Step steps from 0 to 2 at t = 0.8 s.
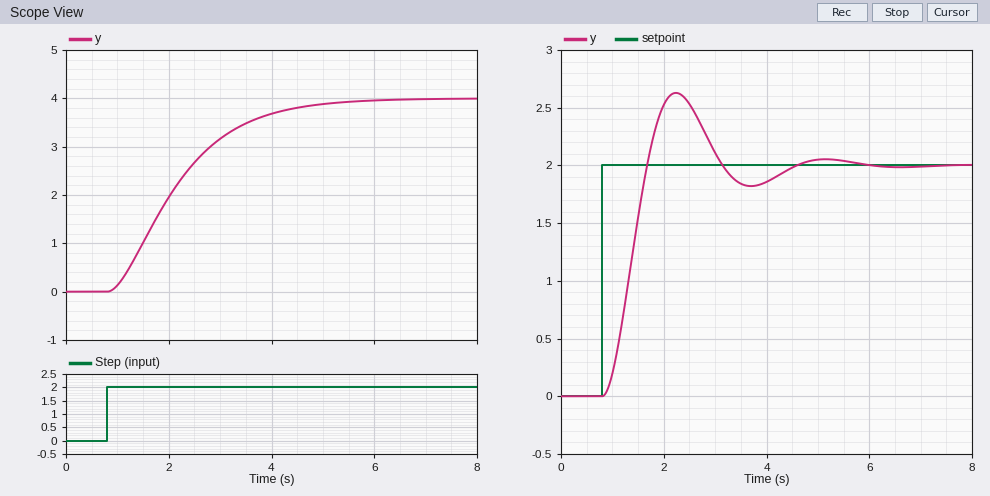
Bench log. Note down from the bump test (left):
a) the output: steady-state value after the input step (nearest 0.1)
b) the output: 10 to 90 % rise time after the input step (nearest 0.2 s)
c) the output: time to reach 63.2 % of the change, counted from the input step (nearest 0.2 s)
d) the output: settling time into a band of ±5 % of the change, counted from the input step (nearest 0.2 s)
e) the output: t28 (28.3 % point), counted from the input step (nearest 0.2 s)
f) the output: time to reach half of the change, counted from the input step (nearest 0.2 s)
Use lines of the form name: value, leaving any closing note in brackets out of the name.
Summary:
the output: steady-state value after the input step: 4.0
the output: 10 to 90 % rise time after the input step: 2.6 s
the output: time to reach 63.2 % of the change, counted from the input step: 1.6 s
the output: settling time into a band of ±5 % of the change, counted from the input step: 3.6 s
the output: t28 (28.3 % point), counted from the input step: 0.8 s
the output: time to reach half of the change, counted from the input step: 1.2 s
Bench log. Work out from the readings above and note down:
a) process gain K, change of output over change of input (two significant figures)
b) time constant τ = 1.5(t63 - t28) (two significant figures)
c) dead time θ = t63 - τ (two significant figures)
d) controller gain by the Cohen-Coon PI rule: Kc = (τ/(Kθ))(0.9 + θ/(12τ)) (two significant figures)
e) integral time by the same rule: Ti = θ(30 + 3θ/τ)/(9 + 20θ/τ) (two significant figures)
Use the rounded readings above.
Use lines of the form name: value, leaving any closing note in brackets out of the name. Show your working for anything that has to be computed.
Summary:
process gain K, change of output over change of input: (4 - 0) / 2 = 2.0
time constant τ = 1.5(t63 - t28): 1.5 × (1.6 - 0.8) = 1.2 s
dead time θ = t63 - τ: 1.6 - 1.2 = 0.40 s
controller gain by the Cohen-Coon PI rule: Kc = (τ/(Kθ))(0.9 + θ/(12τ)): 1.2 / (2 × 0.4) × (0.9 + 0.4 / (12 × 1.2)) = 1.4
integral time by the same rule: Ti = θ(30 + 3θ/τ)/(9 + 20θ/τ): 0.4 × (30 + 3 × 0.4 / 1.2) / (9 + 20 × 0.4 / 1.2) = 0.79 s
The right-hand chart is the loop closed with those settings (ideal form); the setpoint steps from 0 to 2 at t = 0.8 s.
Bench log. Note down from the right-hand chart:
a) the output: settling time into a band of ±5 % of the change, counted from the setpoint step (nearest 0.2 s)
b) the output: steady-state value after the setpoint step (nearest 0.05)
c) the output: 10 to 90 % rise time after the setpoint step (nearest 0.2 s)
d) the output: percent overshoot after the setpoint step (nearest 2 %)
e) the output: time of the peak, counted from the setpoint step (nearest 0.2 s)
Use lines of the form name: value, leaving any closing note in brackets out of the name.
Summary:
the output: settling time into a band of ±5 % of the change, counted from the setpoint step: 3.4 s
the output: steady-state value after the setpoint step: 2.00
the output: 10 to 90 % rise time after the setpoint step: 0.6 s
the output: percent overshoot after the setpoint step: 32 %
the output: time of the peak, counted from the setpoint step: 1.4 s
